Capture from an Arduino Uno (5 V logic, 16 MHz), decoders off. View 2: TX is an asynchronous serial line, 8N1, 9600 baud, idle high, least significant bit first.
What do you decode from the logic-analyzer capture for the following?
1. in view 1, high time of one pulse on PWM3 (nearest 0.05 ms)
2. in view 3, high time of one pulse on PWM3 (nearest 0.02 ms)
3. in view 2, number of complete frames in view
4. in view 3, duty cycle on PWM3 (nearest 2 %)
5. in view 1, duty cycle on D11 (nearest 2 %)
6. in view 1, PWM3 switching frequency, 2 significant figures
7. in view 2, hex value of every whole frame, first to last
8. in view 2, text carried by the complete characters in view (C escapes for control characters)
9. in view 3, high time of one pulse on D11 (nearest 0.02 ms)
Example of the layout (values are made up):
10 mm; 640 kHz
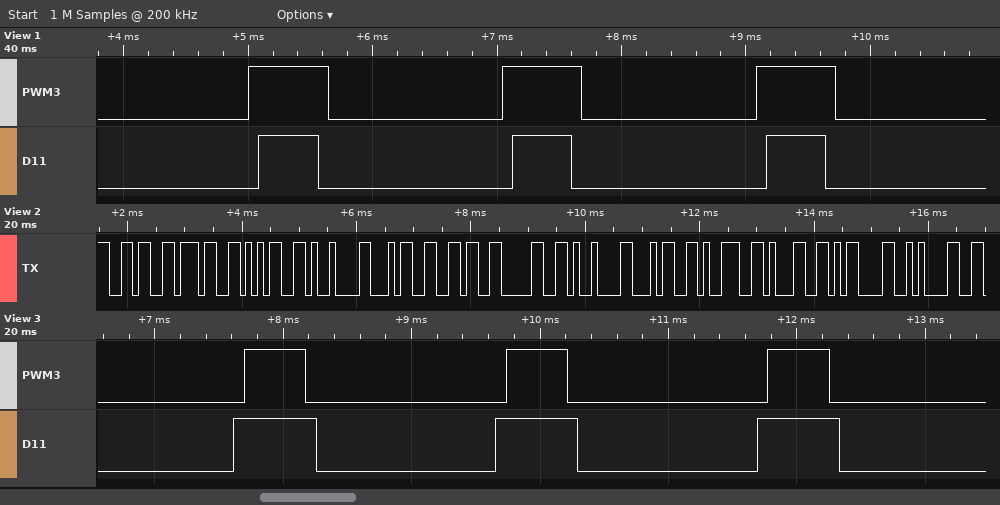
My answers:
0.65 ms; 0.48 ms; 13; 24 %; 24 %; 490 Hz; 36 37 35 09 34 36 30 09 34 39 31 0D 0A; "675\t460\t491\r\n"; 0.64 ms
